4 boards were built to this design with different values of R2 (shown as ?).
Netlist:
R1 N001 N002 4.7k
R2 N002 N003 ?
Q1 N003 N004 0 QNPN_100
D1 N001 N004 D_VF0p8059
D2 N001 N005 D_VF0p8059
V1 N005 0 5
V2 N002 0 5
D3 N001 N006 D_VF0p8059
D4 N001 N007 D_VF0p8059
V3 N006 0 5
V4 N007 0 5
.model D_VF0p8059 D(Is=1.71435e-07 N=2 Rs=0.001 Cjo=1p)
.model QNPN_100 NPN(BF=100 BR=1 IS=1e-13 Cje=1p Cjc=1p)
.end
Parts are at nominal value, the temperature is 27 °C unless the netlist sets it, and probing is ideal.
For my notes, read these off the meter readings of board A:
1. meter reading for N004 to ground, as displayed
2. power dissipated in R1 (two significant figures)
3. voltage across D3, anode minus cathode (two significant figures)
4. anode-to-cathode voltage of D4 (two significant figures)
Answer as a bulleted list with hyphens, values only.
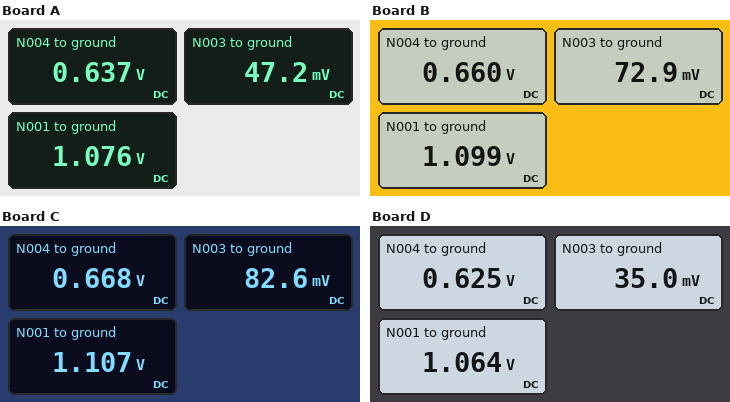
- 0.637 V
- 3.3 mW
- -3.9 V
- -3.9 V
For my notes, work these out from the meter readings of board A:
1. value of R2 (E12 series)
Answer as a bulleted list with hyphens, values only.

- 1.5 kΩ
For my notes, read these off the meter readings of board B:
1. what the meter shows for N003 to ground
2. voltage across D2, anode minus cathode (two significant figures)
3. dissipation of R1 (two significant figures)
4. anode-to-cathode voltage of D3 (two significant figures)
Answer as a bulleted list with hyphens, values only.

- 72.9 mV
- -3.9 V
- 3.2 mW
- -3.9 V
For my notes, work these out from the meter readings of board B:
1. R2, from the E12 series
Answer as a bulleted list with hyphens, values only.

- 470 Ω
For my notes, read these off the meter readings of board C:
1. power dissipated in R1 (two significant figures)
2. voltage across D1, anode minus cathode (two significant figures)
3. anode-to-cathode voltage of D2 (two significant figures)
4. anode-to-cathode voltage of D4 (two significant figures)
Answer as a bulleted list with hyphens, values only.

- 3.2 mW
- 440 mV
- -3.9 V
- -3.9 V
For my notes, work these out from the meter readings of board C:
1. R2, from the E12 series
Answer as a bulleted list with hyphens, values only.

- 330 Ω
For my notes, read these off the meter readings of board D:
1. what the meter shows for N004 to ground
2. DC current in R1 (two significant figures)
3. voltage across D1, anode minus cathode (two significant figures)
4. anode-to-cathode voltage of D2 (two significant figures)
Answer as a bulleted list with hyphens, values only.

- 0.625 V
- 840 µA
- 440 mV
- -3.9 V
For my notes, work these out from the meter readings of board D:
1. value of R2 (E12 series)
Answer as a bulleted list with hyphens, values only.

- 3.3 kΩ
